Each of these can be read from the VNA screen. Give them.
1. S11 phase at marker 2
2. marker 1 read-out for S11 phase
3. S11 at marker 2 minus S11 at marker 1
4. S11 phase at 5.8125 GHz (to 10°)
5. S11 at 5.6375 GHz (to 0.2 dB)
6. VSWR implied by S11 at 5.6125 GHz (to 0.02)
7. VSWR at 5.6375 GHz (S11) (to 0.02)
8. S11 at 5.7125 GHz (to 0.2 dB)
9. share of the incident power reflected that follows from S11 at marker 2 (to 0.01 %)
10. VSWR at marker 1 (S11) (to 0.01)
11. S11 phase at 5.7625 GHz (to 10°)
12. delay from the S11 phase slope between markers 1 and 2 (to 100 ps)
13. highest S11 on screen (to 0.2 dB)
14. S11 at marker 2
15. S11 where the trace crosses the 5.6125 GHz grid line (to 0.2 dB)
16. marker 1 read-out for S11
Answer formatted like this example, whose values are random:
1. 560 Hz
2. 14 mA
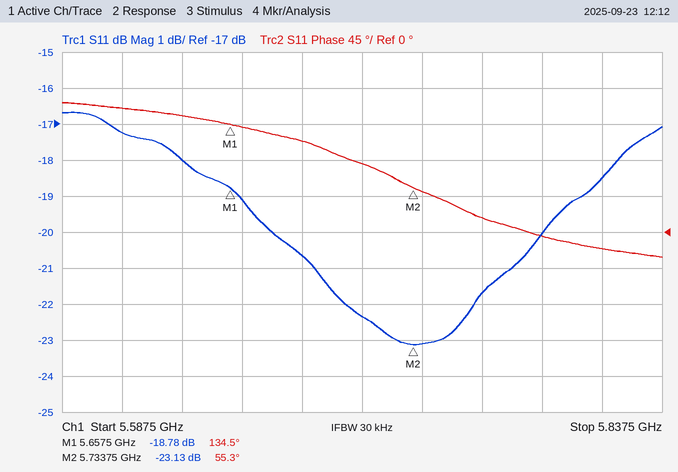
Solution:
1. 55.3°
2. 134.5°
3. -4.35 dB
4. -20°
5. -18.0 dB
6. 1.32
7. 1.28
8. -22.4 dB
9. 0.49 %
10. 1.26
11. 20°
12. 2.9 ns
13. -16.6 dB
14. -23.13 dB
15. -17.2 dB
16. -18.78 dB
